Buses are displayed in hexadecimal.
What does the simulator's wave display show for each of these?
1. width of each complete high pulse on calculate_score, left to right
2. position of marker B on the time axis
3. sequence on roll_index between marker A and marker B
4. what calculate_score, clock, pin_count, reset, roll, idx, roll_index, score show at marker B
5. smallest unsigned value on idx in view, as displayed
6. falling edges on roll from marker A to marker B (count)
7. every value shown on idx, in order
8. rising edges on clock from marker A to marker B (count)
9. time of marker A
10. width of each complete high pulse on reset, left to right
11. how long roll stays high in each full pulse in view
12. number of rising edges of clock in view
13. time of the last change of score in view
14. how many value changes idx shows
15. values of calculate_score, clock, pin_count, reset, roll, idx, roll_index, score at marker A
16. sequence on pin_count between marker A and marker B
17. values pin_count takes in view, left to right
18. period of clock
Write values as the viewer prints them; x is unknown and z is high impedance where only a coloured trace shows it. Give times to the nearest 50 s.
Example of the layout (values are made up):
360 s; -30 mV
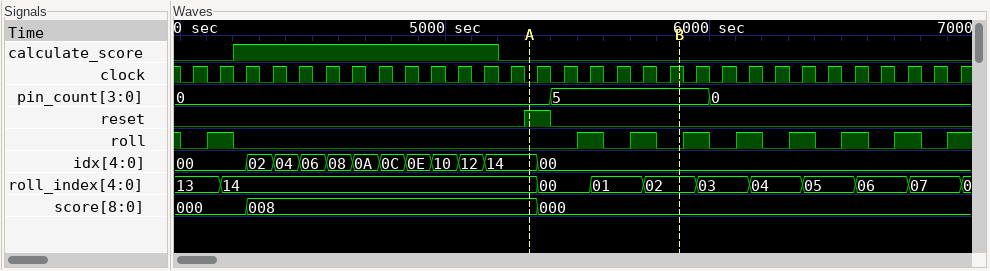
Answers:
1000 s; 5900 s; 14, 00, 01, 02; calculate_score=0, clock=1, pin_count=5, reset=0, roll=0, idx=00, roll_index=02, score=000; 00; 2; 00, 02, 04, 06, 08, 0A, 0C, 0E, 10, 12, 14, 00; 6; 5300 s; 100 s; 100 s, 100 s, 100 s, 100 s, 100 s, 100 s, 100 s, 100 s; 30; 5350 s; 11; calculate_score=0, clock=0, pin_count=0, reset=1, roll=0, idx=14, roll_index=14, score=008; 0, 5; 0, 5, 0; 100 s
